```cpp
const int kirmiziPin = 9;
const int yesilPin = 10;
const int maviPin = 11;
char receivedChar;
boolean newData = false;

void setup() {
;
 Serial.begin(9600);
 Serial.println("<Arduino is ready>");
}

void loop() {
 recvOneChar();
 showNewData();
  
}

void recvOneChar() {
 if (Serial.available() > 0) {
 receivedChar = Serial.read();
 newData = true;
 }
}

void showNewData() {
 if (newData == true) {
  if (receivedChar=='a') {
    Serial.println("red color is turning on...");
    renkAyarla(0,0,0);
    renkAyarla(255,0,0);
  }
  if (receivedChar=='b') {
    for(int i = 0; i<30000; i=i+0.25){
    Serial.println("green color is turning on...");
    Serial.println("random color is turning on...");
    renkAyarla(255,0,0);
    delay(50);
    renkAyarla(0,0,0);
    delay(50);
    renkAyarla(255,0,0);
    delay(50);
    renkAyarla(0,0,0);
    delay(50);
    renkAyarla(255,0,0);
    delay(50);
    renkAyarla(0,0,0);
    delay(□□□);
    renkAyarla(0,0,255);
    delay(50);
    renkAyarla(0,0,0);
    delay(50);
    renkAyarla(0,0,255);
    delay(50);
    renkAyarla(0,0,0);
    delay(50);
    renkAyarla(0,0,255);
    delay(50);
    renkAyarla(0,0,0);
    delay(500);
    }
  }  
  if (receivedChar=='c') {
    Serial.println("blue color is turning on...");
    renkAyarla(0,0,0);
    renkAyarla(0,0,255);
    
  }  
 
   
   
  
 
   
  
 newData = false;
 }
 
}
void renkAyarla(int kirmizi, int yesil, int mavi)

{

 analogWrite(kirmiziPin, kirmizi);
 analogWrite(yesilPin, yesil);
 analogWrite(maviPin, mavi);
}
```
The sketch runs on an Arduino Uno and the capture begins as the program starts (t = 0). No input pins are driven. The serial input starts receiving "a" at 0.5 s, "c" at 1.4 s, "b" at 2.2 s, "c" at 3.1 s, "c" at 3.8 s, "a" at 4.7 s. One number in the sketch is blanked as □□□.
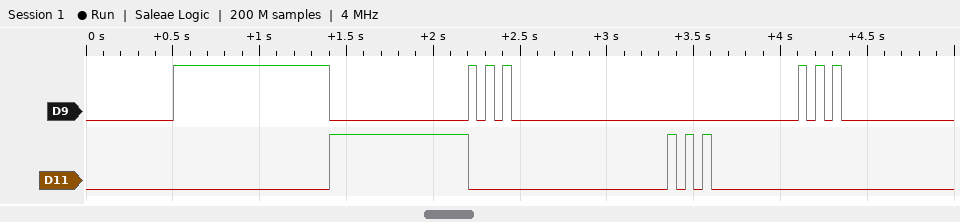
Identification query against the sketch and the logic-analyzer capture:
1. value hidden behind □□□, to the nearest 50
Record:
900
